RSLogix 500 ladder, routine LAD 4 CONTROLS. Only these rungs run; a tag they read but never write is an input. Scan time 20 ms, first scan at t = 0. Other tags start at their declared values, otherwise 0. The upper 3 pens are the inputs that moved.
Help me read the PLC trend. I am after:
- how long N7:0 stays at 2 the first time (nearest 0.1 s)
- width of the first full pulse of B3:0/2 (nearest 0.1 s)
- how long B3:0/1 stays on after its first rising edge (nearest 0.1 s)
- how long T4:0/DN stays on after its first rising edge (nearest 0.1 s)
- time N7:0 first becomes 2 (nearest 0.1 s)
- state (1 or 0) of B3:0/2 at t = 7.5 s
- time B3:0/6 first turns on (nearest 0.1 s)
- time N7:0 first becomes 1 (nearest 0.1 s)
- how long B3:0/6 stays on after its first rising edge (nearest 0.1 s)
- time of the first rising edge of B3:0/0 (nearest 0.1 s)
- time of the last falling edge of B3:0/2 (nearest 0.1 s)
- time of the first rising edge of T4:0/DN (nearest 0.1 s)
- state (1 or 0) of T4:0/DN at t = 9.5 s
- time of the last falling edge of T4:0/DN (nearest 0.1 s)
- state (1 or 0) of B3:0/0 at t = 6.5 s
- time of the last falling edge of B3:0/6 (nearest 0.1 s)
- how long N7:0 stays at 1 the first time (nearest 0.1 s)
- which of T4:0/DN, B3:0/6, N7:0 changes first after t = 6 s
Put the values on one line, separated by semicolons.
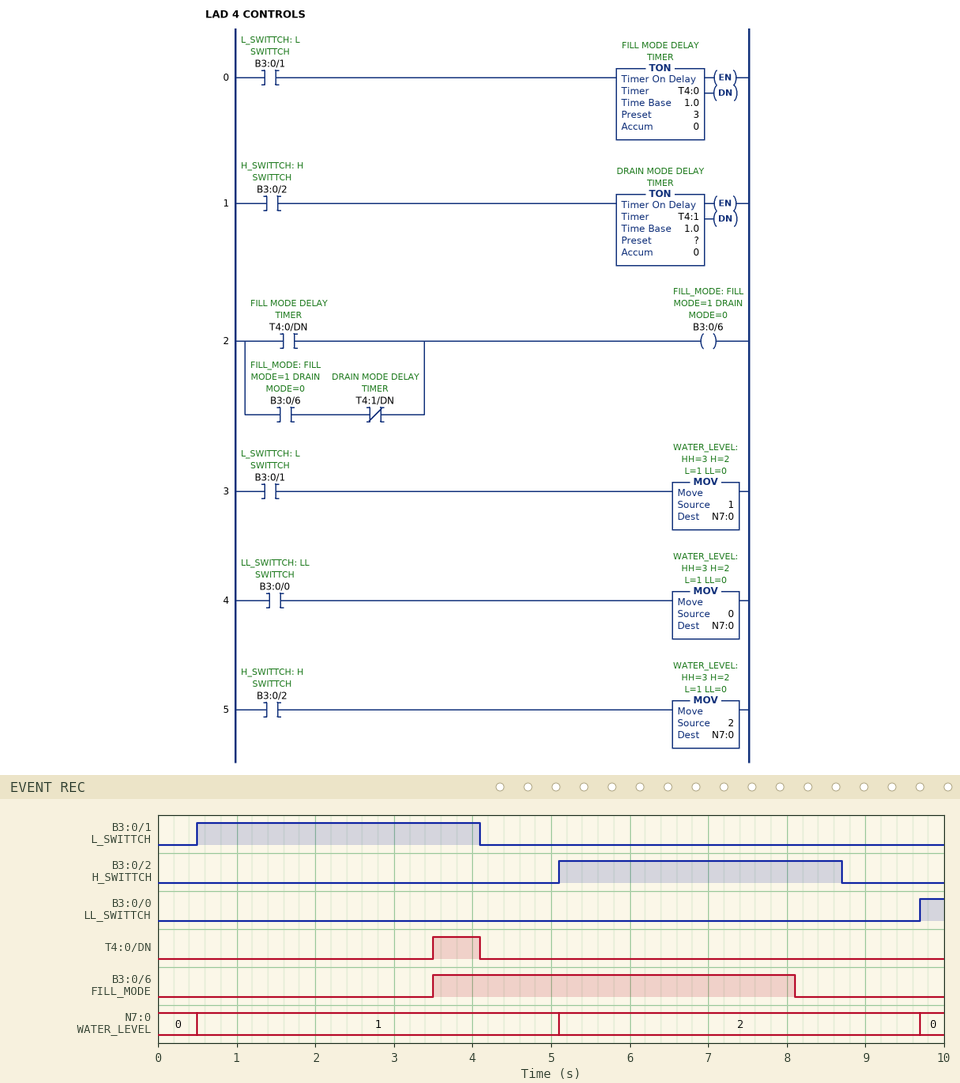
4.6 s; 3.6 s; 3.6 s; 0.6 s; 5.1 s; 1; 3.5 s; 0.5 s; 4.6 s; 9.7 s; 8.7 s; 3.5 s; 0; 4.1 s; 0; 8.1 s; 4.6 s; B3:0/6
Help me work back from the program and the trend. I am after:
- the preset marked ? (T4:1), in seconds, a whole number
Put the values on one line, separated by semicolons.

3 s
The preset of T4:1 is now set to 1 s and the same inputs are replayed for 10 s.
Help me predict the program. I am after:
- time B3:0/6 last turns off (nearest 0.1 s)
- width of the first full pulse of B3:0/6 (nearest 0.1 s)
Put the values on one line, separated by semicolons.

6.1 s; 2.6 s
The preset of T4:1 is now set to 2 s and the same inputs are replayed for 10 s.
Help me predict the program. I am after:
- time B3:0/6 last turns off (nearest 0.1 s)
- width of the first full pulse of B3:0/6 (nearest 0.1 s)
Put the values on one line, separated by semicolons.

7.1 s; 3.6 s
